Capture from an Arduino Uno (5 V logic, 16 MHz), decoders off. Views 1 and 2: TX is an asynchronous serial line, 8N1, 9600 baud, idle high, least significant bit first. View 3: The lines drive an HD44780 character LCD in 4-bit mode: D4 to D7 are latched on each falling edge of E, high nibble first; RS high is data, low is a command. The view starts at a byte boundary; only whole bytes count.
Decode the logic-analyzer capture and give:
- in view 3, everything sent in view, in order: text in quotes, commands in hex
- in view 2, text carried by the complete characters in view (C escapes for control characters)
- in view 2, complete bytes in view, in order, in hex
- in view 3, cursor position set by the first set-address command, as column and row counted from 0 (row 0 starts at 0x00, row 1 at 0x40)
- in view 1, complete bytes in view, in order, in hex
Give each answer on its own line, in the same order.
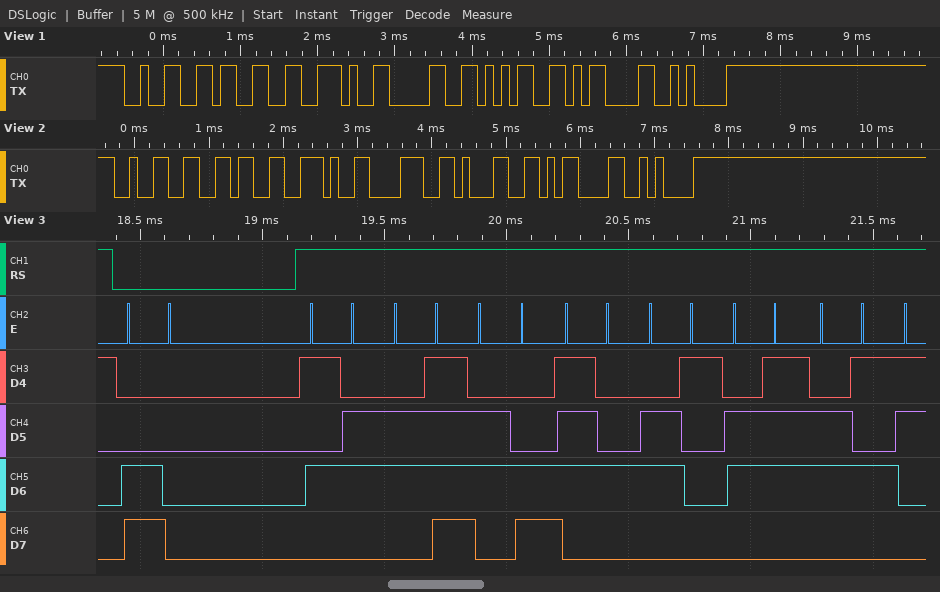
0xC0 "Voltage"
"26.81\r\n"
32 36 2E 38 31 0D 0A
column 0, row 1
32 33 2E 30 35 0D 0A
